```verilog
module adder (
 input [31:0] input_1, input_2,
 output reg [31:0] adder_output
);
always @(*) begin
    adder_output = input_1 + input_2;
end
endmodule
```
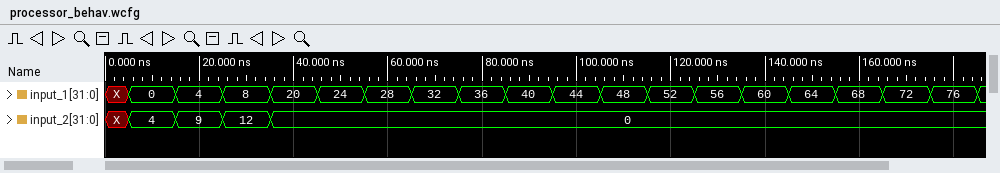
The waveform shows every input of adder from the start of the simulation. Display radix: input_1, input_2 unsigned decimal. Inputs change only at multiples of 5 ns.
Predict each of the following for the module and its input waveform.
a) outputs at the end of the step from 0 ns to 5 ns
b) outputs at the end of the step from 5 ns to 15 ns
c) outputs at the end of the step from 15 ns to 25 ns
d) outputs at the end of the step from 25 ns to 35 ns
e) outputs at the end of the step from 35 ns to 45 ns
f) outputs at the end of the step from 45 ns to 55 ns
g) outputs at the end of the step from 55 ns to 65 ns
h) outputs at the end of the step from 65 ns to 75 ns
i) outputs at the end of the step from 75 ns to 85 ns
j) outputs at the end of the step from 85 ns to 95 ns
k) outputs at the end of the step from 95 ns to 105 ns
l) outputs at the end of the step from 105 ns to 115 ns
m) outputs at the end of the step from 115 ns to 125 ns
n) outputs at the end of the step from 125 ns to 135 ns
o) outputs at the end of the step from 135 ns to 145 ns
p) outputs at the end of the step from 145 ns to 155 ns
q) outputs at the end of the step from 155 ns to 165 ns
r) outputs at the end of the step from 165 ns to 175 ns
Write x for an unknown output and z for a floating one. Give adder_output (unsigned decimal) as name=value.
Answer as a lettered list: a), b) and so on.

a) adder_output=x
b) adder_output=4
c) adder_output=13
d) adder_output=20
e) adder_output=20
f) adder_output=24
g) adder_output=28
h) adder_output=32
i) adder_output=36
j) adder_output=40
k) adder_output=44
l) adder_output=48
m) adder_output=52
n) adder_output=56
o) adder_output=60
p) adder_output=64
q) adder_output=68
r) adder_output=72
